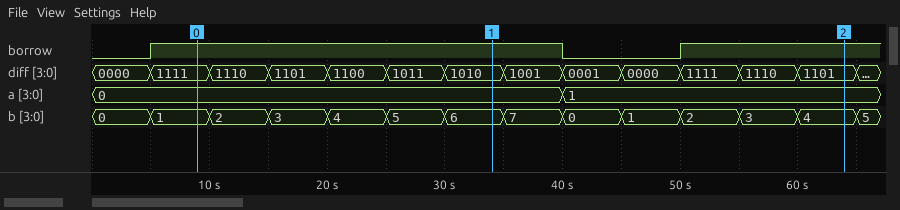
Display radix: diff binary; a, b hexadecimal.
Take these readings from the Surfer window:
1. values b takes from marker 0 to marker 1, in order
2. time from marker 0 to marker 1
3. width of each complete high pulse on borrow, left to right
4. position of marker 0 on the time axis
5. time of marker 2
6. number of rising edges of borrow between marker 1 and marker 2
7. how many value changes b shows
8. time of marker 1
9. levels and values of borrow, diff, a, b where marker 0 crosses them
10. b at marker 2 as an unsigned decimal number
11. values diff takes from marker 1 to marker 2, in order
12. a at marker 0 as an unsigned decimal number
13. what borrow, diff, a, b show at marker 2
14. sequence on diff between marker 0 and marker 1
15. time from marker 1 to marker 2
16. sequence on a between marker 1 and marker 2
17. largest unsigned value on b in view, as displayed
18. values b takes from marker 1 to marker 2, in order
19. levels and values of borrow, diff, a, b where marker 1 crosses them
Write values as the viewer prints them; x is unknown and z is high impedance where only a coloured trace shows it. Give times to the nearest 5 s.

1, 2, 3, 4, 5, 6
25 s
35 s
10 s
65 s
1
13
35 s
borrow=1, diff=1111, a=0, b=1
4
1010, 1001, 0001, 0000, 1111, 1110, 1101
0
borrow=1, diff=1101, a=1, b=4
1111, 1110, 1101, 1100, 1011, 1010
30 s
0, 1
7
6, 7, 0, 1, 2, 3, 4
borrow=1, diff=1010, a=0, b=6
